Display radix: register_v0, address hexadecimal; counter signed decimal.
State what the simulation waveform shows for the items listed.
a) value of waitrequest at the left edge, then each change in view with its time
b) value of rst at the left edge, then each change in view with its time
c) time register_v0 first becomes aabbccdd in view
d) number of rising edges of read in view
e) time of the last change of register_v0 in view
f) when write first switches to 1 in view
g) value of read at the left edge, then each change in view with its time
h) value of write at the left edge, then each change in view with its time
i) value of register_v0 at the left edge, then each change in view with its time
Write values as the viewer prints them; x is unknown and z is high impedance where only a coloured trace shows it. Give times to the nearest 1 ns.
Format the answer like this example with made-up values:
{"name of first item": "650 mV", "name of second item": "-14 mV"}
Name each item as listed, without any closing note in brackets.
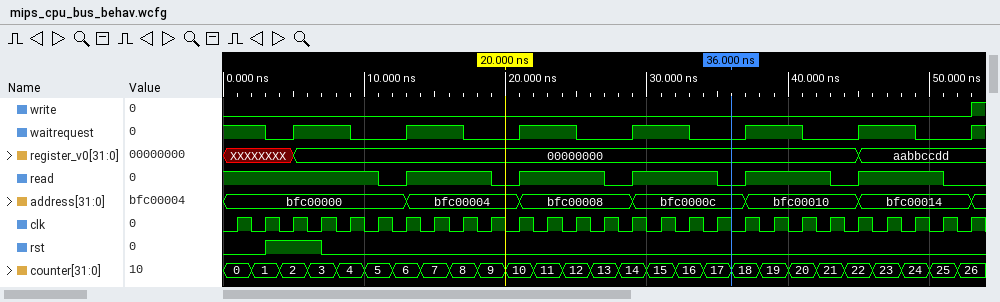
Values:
{"value of waitrequest at the left edge, then each change in view with its time": "1, 0 at 3 ns, 1 at 5 ns, 0 at 9 ns, 1 at 13 ns, 0 at 17 ns, 1 at 21 ns, 0 at 25 ns, 1 at 29 ns, 0 at 33 ns, 1 at 37 ns, 0 at 41 ns, 1 at 45 ns, 0 at 49 ns, 1 at 53 ns", "value of rst at the left edge, then each change in view with its time": "0, 1 at 3 ns, 0 at 7 ns", "time register_v0 first becomes aabbccdd in view": "45 ns", "number of rising edges of read in view": "5", "time of the last change of register_v0 in view": "45 ns", "when write first switches to 1 in view": "53 ns", "value of read at the left edge, then each change in view with its time": "1, 0 at 11 ns, 1 at 13 ns, 0 at 19 ns, 1 at 21 ns, 0 at 27 ns, 1 at 29 ns, 0 at 35 ns, 1 at 37 ns, 0 at 43 ns, 1 at 45 ns, 0 at 51 ns", "value of write at the left edge, then each change in view with its time": "0, 1 at 53 ns", "value of register_v0 at the left edge, then each change in view with its time": "XXXXXXXX, 00000000 at 5 ns, aabbccdd at 45 ns"}
